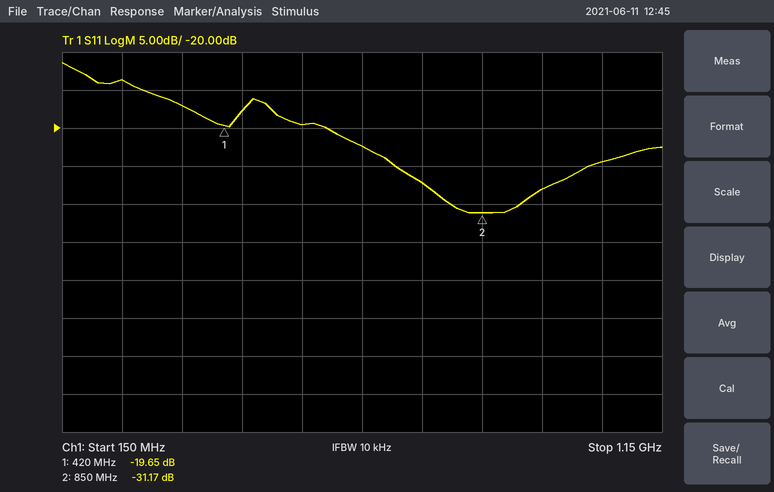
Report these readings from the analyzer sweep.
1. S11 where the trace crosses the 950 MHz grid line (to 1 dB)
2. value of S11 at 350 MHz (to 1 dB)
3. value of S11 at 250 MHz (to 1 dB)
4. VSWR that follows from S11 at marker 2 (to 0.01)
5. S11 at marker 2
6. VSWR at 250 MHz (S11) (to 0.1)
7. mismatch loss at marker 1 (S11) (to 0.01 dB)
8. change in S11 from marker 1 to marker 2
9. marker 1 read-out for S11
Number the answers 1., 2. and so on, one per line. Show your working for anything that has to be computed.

1. -28 dB
2. -17 dB
3. -14 dB
4. (1 + 0.0276)/(1 − 0.0276) ≈ 1.06
5. -31.17 dB
6. |Γ| = 10^(-14/20) = 0.1995; VSWR = (1 + 0.1995)/(1 − 0.1995) ≈ 1.5
7. −10 log10(1 − 10^(-19.65/10)) ≈ 0.05 dB
8. -31.17 − (-19.65) = -11.52 dB
9. -19.65 dB
